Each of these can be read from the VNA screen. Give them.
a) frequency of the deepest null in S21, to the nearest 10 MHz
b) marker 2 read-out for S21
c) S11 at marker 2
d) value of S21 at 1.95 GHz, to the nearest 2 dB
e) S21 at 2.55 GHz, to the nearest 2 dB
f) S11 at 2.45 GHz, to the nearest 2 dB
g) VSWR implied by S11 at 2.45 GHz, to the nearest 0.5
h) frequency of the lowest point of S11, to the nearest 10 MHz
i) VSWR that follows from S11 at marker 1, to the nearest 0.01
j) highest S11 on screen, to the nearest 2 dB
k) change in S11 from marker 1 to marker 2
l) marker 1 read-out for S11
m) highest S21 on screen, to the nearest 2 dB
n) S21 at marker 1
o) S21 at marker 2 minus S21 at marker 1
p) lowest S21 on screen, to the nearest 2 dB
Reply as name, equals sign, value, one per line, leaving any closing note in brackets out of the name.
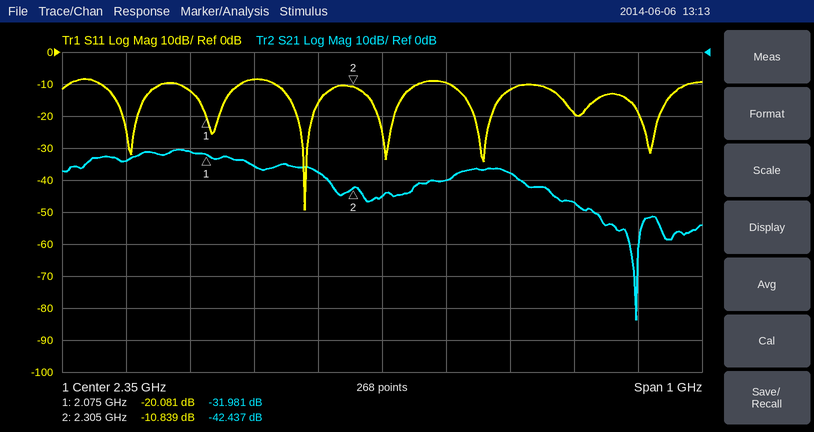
frequency of the deepest null in S21, to the nearest 10 MHz = 2.75 GHz
marker 2 read-out for S21 = -42.437 dB
S11 at marker 2 = -10.839 dB
value of S21 at 1.95 GHz, to the nearest 2 dB = -34 dB
S21 at 2.55 GHz, to the nearest 2 dB = -38 dB
S11 at 2.45 GHz, to the nearest 2 dB = -10 dB
VSWR implied by S11 at 2.45 GHz, to the nearest 0.5 = 2.0
frequency of the lowest point of S11, to the nearest 10 MHz = 2.23 GHz
VSWR that follows from S11 at marker 1, to the nearest 0.01 = 1.22
highest S11 on screen, to the nearest 2 dB = -8 dB
change in S11 from marker 1 to marker 2 = 9.242 dB
marker 1 read-out for S11 = -20.081 dB
highest S21 on screen, to the nearest 2 dB = -30 dB
S21 at marker 1 = -31.981 dB
S21 at marker 2 minus S21 at marker 1 = -10.456 dB
lowest S21 on screen, to the nearest 2 dB = -84 dB
